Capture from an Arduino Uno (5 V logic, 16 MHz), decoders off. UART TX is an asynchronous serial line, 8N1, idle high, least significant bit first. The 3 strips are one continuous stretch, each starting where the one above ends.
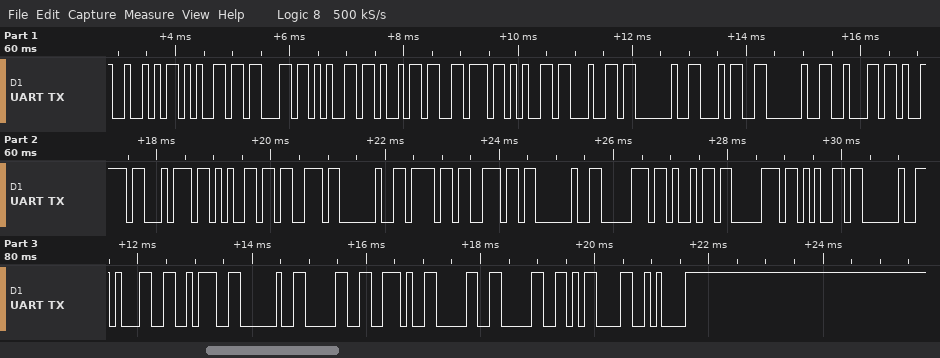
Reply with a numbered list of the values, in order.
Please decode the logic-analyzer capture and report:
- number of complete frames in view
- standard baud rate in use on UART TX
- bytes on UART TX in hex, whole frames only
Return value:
1. 34
2. 9600 baud
3. 52 65 63 65 69 76 65 64 20 34 20 62 79 74 65 73 20 6F 6E 20 70 69 70 65 20 31 3A 20 30 2E 30 30 0D 0A
